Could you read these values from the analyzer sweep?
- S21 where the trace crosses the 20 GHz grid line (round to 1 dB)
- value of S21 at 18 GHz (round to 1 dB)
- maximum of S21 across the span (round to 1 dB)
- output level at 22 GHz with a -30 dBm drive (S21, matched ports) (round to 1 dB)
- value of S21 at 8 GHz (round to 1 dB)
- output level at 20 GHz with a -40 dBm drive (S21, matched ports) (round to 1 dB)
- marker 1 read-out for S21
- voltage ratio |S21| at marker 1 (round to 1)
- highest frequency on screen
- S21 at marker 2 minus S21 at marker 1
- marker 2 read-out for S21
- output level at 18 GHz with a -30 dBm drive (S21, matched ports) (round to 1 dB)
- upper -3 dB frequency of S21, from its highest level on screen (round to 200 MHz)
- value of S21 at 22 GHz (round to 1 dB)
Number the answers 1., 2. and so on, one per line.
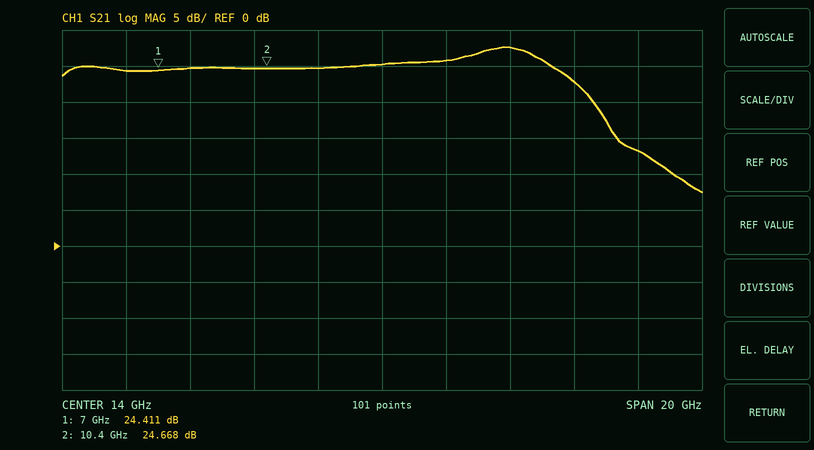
1. 23 dB
2. 28 dB
3. 28 dB
4. -17 dBm
5. 25 dB
6. -17 dBm
7. 24.411 dB
8. 17
9. 24 GHz
10. 0.257 dB
11. 24.668 dB
12. -2 dBm
13. 19.4 GHz
14. 13 dB
